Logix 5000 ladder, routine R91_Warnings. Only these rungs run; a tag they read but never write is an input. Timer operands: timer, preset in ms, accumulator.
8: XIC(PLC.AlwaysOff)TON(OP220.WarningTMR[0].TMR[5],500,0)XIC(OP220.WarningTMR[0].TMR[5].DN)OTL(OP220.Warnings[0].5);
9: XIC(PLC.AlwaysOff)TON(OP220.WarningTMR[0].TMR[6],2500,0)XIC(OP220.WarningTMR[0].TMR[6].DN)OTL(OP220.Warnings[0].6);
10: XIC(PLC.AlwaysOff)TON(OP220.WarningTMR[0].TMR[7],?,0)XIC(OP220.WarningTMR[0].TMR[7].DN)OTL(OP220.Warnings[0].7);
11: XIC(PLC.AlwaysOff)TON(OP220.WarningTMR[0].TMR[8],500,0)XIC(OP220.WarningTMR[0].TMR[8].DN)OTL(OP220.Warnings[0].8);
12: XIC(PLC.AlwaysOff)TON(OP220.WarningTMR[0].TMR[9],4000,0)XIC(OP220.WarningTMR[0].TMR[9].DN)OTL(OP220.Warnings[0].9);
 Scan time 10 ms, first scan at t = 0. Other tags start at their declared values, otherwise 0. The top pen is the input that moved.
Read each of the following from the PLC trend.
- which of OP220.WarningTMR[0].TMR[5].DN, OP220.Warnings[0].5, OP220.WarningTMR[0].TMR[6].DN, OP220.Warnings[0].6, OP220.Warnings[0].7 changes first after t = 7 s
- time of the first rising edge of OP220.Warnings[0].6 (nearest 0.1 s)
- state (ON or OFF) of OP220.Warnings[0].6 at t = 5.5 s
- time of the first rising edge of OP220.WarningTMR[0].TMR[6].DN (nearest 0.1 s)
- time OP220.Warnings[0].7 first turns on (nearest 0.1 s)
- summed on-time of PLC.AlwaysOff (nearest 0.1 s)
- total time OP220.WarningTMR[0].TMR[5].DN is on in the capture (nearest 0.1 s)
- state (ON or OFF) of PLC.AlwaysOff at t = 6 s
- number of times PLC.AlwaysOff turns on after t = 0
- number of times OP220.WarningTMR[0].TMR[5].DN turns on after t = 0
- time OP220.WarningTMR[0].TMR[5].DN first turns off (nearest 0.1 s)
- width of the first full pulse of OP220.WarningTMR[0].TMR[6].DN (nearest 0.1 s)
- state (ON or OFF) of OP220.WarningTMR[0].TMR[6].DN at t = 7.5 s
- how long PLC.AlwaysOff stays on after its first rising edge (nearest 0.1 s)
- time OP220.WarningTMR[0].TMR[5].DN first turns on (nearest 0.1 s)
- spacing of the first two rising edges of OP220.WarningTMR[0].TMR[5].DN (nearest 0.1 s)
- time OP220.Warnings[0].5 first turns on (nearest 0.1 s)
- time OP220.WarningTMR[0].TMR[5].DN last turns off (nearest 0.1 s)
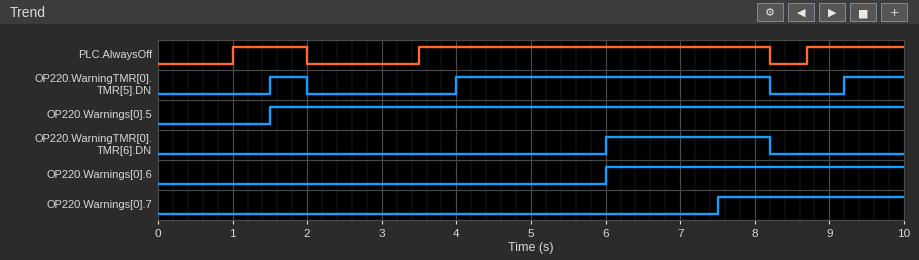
OP220.Warnings[0].7
6.0 s
OFF
6.0 s
7.5 s
7.0 s
5.5 s
ON
3
3
2.0 s
2.2 s
ON
1.0 s
1.5 s
2.5 s
1.5 s
8.2 s
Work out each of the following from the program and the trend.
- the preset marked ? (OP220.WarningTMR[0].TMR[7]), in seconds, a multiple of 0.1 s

4.0 s
